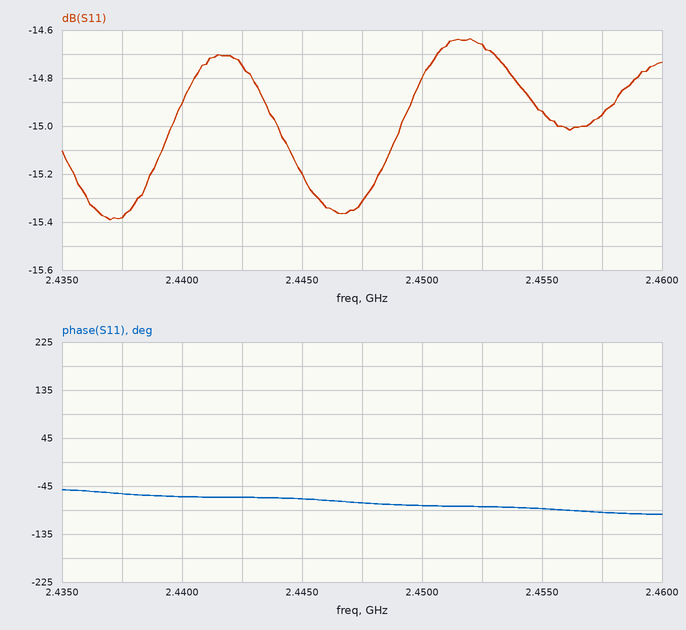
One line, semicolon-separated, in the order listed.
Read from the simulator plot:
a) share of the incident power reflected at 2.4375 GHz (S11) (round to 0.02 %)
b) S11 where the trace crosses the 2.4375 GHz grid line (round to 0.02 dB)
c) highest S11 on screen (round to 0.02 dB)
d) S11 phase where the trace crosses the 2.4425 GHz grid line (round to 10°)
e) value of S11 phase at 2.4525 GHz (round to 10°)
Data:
2.90 %; -15.38 dB; -14.64 dB; -70°; -80°
